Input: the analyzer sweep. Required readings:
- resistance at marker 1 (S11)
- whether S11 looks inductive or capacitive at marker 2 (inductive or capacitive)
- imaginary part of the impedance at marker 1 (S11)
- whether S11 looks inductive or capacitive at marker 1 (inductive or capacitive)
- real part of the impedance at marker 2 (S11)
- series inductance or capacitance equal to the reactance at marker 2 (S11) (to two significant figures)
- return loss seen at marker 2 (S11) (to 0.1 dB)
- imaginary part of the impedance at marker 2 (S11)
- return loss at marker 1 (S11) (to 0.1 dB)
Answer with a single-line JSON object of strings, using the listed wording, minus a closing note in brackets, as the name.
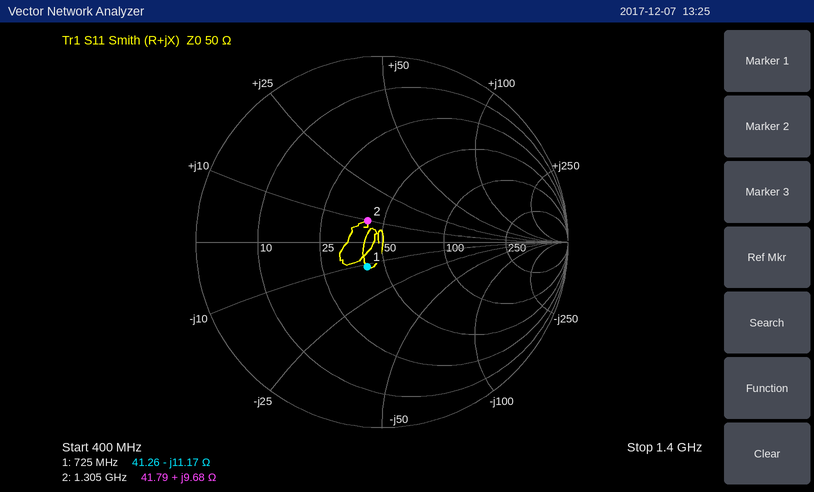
{"resistance at marker 1": "41.26 Ω", "whether S11 looks inductive or capacitive at marker 2": "inductive", "imaginary part of the impedance at marker 1": "-11.17 Ω", "whether S11 looks inductive or capacitive at marker 1": "capacitive", "real part of the impedance at marker 2": "41.79 Ω", "series inductance or capacitance equal to the reactance at marker 2 (S11)": "1.2 nH", "return loss seen at marker 2 (S11)": "17.2 dB", "imaginary part of the impedance at marker 2": "+9.68 Ω", "return loss at marker 1 (S11)": "16.2 dB"}
